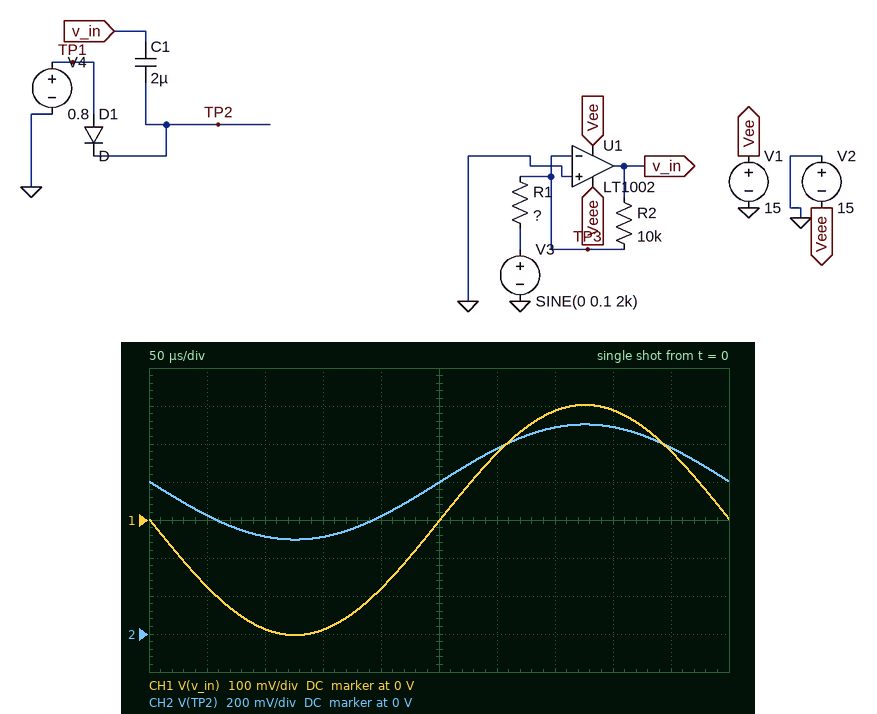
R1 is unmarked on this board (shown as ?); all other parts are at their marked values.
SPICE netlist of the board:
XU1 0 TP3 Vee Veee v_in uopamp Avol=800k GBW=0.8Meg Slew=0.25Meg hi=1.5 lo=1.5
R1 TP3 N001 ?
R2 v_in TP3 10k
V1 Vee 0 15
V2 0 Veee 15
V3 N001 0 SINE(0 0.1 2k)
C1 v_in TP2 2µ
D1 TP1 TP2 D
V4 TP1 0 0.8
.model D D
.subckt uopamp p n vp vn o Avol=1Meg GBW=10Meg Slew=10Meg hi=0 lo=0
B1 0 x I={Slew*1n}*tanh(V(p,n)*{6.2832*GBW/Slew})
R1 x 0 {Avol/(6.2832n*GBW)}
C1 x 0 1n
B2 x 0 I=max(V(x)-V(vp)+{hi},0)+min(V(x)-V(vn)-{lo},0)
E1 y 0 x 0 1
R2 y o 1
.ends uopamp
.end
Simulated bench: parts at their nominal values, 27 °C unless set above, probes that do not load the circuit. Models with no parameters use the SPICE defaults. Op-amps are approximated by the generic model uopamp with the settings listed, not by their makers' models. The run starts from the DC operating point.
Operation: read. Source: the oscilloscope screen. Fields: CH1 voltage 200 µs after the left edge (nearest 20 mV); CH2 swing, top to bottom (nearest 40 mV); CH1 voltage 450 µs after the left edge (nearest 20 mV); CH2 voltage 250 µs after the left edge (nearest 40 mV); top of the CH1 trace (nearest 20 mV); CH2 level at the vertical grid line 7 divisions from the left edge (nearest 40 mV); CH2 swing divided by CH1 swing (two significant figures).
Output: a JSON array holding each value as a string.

["-180 mV", "600 mV", "180 mV", "800 mV", "300 mV", "1.08 V", "1.0"]
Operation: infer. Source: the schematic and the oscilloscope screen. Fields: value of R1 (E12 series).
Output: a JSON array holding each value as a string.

["3.3 kΩ"]
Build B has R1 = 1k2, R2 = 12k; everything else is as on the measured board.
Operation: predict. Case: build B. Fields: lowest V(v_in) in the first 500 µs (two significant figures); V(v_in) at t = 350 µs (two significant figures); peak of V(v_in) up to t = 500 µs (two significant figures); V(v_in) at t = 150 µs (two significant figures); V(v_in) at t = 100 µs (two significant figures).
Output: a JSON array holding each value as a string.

["-1.0 V", "940 mV", "1.0 V", "-960 mV", "-940 mV"]
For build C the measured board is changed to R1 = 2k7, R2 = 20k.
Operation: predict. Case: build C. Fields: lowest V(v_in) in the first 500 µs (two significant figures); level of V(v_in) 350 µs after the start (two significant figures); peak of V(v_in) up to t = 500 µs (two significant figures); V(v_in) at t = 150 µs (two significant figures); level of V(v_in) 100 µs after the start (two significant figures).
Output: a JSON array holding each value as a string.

["-740 mV", "700 mV", "740 mV", "-710 mV", "-700 mV"]
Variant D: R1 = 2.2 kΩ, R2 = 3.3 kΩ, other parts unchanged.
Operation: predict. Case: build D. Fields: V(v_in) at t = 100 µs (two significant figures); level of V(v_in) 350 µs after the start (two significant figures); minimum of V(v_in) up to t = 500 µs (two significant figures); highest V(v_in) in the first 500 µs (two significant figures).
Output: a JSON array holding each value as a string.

["-140 mV", "140 mV", "-150 mV", "150 mV"]
